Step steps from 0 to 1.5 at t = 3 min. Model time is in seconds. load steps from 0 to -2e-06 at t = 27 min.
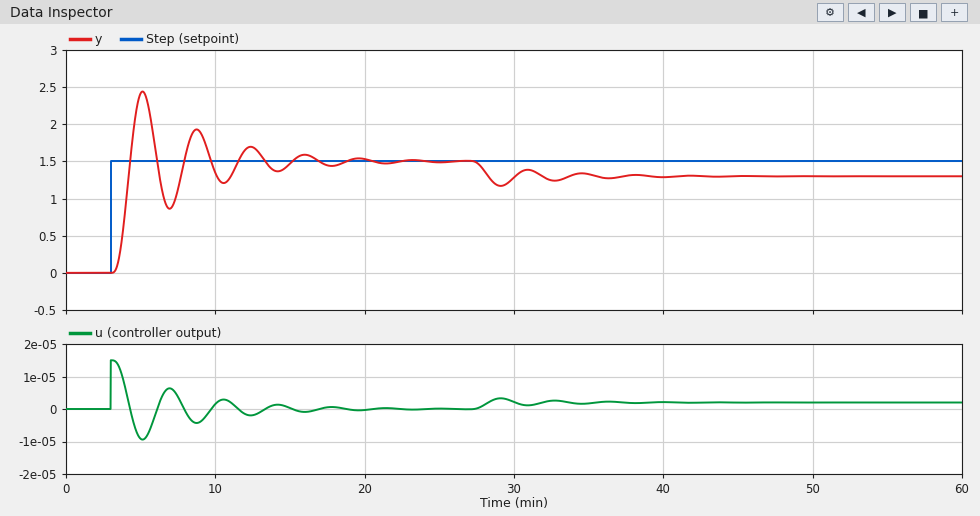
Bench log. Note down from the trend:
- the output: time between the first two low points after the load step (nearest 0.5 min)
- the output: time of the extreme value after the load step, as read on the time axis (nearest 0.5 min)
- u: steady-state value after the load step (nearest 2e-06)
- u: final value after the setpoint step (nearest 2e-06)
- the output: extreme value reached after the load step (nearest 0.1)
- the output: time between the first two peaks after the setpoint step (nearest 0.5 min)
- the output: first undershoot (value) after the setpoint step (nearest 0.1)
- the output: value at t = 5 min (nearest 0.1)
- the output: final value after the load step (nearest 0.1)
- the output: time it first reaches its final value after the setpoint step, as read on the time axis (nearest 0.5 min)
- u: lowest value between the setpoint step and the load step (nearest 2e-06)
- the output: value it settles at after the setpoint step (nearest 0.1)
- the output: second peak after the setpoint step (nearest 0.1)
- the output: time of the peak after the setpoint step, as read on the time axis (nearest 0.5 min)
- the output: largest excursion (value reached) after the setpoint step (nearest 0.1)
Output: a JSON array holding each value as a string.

["3.5 min", "29.0 min", "0.000002", "0.000000", "1.2", "3.5 min", "0.9", "2.4", "1.3", "4.5 min", "-0.000010", "1.5", "1.9", "5.0 min", "2.4"]
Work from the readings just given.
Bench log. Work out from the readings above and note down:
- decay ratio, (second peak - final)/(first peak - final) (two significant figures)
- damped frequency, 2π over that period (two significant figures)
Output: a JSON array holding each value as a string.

["0.44", "1.8 rad/min"]
